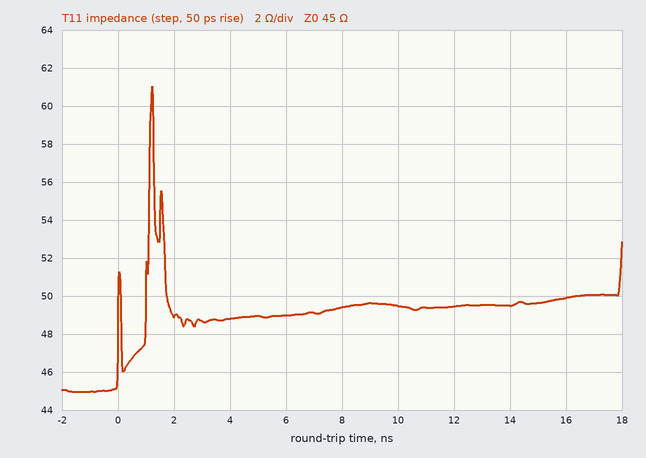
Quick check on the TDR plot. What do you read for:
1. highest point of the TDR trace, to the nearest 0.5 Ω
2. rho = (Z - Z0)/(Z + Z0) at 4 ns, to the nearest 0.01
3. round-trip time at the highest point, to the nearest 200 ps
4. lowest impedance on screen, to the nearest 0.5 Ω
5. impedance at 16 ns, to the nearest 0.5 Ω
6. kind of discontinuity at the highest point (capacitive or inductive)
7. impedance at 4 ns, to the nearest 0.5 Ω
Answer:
61.0 Ω
+0.04
1.2 ns
45.0 Ω
50.0 Ω
inductive
49.0 Ω
